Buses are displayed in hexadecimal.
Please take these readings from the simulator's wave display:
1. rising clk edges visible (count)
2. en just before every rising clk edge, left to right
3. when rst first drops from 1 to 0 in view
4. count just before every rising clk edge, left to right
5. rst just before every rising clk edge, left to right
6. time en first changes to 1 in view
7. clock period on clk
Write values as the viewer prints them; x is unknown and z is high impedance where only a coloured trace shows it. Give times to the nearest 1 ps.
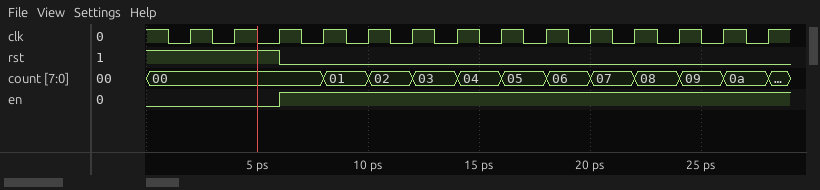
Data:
14
0 0 0 1 1 1 1 1 1 1 1 1 1 1
6 ps
00, 00, 00, 00, 01, 02, 03, 04, 05, 06, 07, 08, 09, 0a
1 1 1 0 0 0 0 0 0 0 0 0 0 0
6 ps
2 ps
